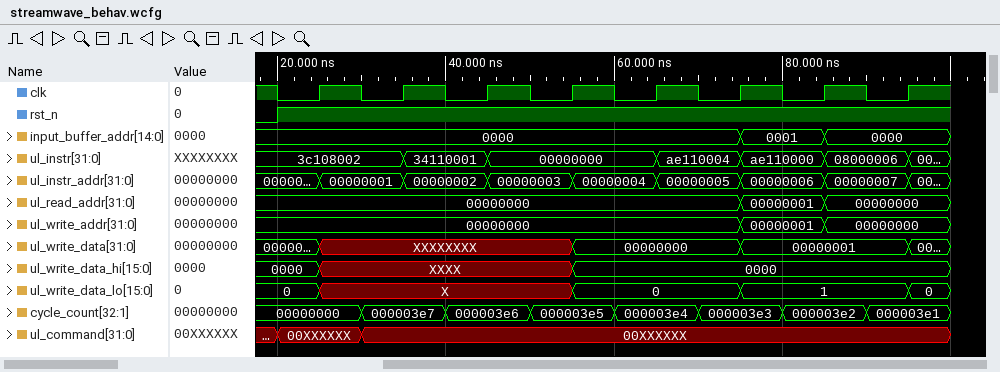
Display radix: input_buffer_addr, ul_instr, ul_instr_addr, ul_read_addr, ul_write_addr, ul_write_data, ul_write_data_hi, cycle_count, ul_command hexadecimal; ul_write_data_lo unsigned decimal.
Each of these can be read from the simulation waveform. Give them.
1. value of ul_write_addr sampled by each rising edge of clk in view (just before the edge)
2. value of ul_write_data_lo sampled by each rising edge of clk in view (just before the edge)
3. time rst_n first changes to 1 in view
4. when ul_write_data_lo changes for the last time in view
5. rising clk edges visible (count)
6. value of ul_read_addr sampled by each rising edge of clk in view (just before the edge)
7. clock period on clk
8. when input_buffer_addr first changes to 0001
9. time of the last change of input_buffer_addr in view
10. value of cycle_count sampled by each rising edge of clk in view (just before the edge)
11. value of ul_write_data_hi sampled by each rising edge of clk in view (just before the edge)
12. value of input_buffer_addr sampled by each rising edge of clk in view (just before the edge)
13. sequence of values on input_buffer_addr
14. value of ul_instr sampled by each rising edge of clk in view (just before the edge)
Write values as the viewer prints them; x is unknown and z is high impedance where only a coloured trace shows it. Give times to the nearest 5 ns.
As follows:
00000000, 00000000, 00000000, 00000000, 00000000, 00000000, 00000001, 00000000
0, X, X, X, 0, 0, 1, 1
20 ns
95 ns
8
00000000, 00000000, 00000000, 00000000, 00000000, 00000000, 00000001, 00000000
10 ns
75 ns
85 ns
00000000, 000003e7, 000003e6, 000003e5, 000003e4, 000003e3, 000003e2, 000003e1
0000, XXXX, XXXX, XXXX, 0000, 0000, 0000, 0000
0000, 0000, 0000, 0000, 0000, 0000, 0001, 0000
0000, 0001, 0000
3c108002, 3c108002, 34110001, 00000000, 00000000, ae110004, ae110000, 08000006
